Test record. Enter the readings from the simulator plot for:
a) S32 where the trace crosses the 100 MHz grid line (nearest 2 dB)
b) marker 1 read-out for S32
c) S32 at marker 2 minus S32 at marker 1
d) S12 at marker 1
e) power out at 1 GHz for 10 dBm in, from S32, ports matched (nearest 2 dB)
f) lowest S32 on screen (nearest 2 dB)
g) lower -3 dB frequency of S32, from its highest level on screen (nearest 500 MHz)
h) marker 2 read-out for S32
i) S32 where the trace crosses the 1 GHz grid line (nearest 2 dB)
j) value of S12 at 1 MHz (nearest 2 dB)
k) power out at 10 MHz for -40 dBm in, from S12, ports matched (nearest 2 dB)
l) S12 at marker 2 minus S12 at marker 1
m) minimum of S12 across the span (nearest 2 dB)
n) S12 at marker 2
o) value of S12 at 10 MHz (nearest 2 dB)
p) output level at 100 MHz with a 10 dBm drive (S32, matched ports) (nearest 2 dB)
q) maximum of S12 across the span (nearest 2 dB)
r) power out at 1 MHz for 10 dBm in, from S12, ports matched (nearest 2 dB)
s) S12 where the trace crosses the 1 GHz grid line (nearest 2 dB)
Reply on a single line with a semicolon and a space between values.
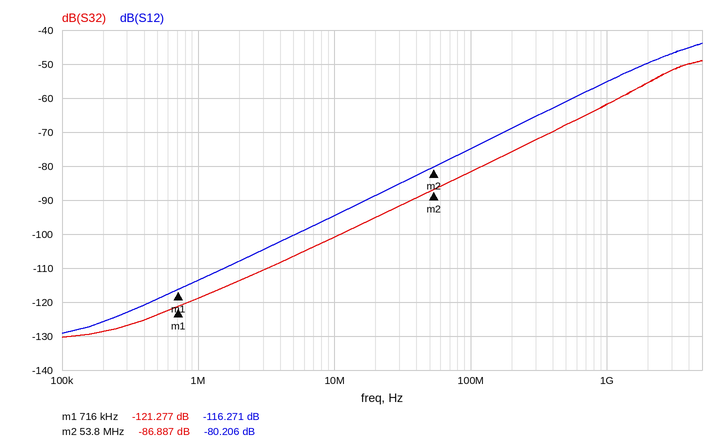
-82 dB; -121.277 dB; 34.390 dB; -116.271 dB; -52 dBm; -130 dB; 3.0 GHz; -86.887 dB; -62 dB; -114 dB; -134 dBm; 36.065 dB; -130 dB; -80.206 dB; -94 dB; -72 dBm; -44 dB; -104 dBm; -56 dB
